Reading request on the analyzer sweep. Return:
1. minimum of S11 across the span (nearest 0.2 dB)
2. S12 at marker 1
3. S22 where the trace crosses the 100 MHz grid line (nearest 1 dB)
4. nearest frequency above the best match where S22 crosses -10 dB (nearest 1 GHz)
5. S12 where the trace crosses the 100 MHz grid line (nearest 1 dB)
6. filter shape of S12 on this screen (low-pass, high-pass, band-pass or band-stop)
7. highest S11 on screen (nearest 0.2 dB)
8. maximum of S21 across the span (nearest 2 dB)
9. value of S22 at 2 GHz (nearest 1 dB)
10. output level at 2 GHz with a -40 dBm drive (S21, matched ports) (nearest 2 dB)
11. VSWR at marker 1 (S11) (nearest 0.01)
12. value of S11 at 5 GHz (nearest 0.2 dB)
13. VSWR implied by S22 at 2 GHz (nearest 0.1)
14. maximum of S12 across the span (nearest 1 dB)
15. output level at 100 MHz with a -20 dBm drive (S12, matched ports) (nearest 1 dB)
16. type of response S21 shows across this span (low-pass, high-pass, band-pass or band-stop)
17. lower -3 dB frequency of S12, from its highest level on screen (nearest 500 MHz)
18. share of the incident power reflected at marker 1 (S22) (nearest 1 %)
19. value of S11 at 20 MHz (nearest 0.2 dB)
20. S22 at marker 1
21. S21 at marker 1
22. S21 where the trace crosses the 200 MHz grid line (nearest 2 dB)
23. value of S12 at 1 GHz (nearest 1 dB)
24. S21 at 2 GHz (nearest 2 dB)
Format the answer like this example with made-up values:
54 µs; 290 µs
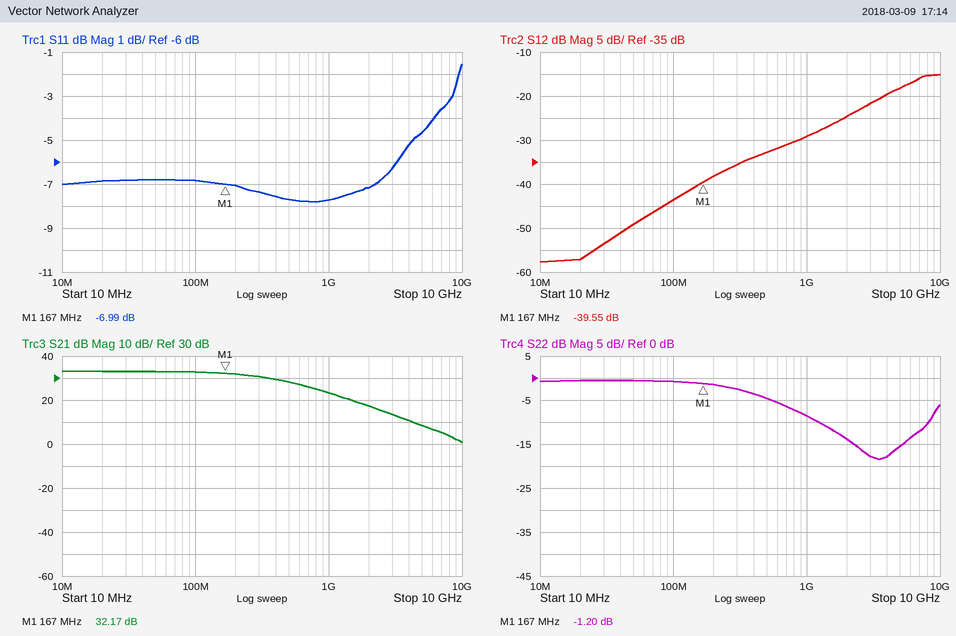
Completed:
-7.8 dB; -39.55 dB; -1 dB; 8 GHz; -44 dB; high-pass; -1.6 dB; 34 dB; -14 dB; -22 dBm; 2.62; -4.6 dB; 1.5; -15 dB; -64 dBm; low-pass; 5.0 GHz; 76 %; -6.8 dB; -1.20 dB; 32.17 dB; 32 dB; -29 dB; 18 dB
